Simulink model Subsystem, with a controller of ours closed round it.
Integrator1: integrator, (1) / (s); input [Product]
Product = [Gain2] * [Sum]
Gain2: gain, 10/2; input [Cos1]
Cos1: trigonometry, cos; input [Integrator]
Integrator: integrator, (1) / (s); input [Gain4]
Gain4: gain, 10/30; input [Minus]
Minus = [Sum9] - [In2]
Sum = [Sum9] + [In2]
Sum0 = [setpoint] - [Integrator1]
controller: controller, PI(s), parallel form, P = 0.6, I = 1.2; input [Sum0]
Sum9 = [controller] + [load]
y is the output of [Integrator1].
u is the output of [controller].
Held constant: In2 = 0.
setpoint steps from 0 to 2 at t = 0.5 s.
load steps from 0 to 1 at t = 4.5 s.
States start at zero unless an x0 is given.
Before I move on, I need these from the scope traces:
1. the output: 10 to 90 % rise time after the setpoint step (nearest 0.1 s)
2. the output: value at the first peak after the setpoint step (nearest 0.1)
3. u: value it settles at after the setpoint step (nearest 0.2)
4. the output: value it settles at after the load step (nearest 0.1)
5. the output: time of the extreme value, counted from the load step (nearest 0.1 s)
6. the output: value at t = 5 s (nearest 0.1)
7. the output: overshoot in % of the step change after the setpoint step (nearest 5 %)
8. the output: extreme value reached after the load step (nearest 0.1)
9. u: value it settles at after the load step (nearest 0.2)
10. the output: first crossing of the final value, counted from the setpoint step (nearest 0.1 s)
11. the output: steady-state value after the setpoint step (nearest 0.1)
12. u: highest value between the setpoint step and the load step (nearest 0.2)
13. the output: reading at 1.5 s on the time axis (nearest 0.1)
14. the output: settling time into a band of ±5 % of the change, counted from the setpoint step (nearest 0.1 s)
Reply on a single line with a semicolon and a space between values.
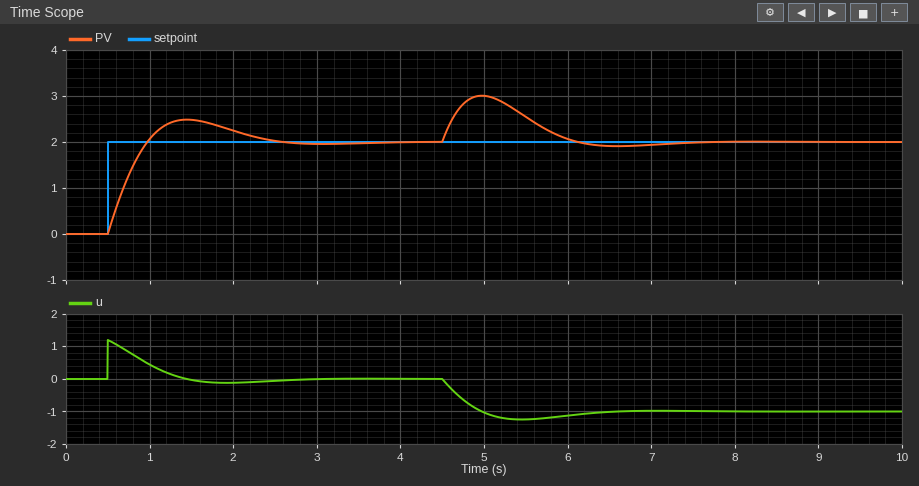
0.4 s; 2.5; 0.0; 2.0; 0.5 s; 3.0; 25 %; 3.0; -1.0; 0.5 s; 2.0; 1.2; 2.5; 1.8 s
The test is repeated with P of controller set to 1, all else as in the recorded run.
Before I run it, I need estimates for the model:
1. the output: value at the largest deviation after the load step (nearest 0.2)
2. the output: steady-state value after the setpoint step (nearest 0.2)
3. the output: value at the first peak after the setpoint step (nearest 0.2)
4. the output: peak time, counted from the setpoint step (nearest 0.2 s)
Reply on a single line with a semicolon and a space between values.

2.8; 2.0; 2.2; 0.8 s
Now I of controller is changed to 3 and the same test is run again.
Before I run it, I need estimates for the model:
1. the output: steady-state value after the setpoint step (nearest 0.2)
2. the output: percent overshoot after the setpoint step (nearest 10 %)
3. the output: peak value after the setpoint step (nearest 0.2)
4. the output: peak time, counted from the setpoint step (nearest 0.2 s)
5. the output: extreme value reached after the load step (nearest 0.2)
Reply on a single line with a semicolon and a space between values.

2.0; 40 %; 2.8; 0.6 s; 2.8
